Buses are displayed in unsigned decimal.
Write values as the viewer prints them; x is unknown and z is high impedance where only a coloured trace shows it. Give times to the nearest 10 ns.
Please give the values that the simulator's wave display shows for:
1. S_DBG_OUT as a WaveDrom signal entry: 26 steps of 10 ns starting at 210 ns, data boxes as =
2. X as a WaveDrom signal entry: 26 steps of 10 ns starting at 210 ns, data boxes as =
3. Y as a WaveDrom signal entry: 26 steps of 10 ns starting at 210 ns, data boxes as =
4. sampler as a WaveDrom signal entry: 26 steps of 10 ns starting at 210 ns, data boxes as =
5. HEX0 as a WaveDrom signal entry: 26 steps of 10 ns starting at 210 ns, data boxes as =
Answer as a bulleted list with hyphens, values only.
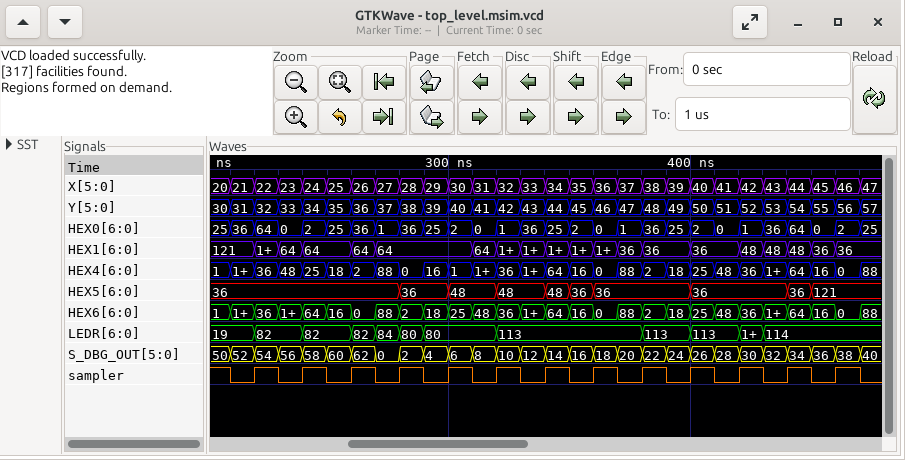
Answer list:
- {name: 'S_DBG_OUT', wave: '==========================', data: '52 54 56 58 60 62 0 2 4 6 8 10 12 14 16 18 20 22 24 26 28 30 32 34 36 38'}
- {name: 'X', wave: '==========================', data: '21 22 23 24 25 26 27 28 29 30 31 32 33 34 35 36 37 38 39 40 41 42 43 44 45 46'}
- {name: 'Y', wave: '==========================', data: '31 32 33 34 35 36 37 38 39 40 41 42 43 44 45 46 47 48 49 50 51 52 53 54 55 56'}
- {name: 'sampler', wave: '01010101010101010101010101'}
- {name: 'HEX0', wave: '==========================', data: '36 64 0 2 25 36 1 36 25 2 0 1 36 25 2 0 1 36 25 2 0 1 36 64 0 2'}
